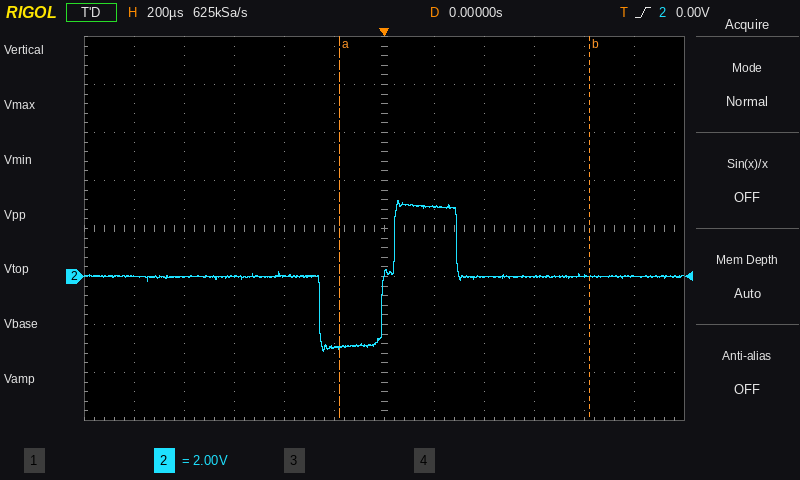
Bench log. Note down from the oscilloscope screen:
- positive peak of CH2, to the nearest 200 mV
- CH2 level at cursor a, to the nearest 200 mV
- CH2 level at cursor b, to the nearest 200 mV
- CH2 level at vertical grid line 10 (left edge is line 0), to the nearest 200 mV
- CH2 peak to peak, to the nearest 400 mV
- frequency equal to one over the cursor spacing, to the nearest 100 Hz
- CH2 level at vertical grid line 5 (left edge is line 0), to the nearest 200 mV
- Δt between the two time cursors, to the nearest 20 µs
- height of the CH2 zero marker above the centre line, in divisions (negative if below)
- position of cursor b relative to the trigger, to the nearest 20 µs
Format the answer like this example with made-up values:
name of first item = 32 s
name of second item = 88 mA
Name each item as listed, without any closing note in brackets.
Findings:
positive peak of CH2, to the nearest 200 mV = 3.2 V
CH2 level at cursor a, to the nearest 200 mV = -3.0 V
CH2 level at cursor b, to the nearest 200 mV = 0.0 V
CH2 level at vertical grid line 10 (left edge is line 0), to the nearest 200 mV = 0.0 V
CH2 peak to peak, to the nearest 400 mV = 6.4 V
frequency equal to one over the cursor spacing, to the nearest 100 Hz = 1.0 kHz
CH2 level at vertical grid line 5 (left edge is line 0), to the nearest 200 mV = -3.0 V
Δt between the two time cursors, to the nearest 20 µs = 1.00 ms
height of the CH2 zero marker above the centre line, in divisions = -1.0 div
position of cursor b relative to the trigger, to the nearest 20 µs = +820 µs
